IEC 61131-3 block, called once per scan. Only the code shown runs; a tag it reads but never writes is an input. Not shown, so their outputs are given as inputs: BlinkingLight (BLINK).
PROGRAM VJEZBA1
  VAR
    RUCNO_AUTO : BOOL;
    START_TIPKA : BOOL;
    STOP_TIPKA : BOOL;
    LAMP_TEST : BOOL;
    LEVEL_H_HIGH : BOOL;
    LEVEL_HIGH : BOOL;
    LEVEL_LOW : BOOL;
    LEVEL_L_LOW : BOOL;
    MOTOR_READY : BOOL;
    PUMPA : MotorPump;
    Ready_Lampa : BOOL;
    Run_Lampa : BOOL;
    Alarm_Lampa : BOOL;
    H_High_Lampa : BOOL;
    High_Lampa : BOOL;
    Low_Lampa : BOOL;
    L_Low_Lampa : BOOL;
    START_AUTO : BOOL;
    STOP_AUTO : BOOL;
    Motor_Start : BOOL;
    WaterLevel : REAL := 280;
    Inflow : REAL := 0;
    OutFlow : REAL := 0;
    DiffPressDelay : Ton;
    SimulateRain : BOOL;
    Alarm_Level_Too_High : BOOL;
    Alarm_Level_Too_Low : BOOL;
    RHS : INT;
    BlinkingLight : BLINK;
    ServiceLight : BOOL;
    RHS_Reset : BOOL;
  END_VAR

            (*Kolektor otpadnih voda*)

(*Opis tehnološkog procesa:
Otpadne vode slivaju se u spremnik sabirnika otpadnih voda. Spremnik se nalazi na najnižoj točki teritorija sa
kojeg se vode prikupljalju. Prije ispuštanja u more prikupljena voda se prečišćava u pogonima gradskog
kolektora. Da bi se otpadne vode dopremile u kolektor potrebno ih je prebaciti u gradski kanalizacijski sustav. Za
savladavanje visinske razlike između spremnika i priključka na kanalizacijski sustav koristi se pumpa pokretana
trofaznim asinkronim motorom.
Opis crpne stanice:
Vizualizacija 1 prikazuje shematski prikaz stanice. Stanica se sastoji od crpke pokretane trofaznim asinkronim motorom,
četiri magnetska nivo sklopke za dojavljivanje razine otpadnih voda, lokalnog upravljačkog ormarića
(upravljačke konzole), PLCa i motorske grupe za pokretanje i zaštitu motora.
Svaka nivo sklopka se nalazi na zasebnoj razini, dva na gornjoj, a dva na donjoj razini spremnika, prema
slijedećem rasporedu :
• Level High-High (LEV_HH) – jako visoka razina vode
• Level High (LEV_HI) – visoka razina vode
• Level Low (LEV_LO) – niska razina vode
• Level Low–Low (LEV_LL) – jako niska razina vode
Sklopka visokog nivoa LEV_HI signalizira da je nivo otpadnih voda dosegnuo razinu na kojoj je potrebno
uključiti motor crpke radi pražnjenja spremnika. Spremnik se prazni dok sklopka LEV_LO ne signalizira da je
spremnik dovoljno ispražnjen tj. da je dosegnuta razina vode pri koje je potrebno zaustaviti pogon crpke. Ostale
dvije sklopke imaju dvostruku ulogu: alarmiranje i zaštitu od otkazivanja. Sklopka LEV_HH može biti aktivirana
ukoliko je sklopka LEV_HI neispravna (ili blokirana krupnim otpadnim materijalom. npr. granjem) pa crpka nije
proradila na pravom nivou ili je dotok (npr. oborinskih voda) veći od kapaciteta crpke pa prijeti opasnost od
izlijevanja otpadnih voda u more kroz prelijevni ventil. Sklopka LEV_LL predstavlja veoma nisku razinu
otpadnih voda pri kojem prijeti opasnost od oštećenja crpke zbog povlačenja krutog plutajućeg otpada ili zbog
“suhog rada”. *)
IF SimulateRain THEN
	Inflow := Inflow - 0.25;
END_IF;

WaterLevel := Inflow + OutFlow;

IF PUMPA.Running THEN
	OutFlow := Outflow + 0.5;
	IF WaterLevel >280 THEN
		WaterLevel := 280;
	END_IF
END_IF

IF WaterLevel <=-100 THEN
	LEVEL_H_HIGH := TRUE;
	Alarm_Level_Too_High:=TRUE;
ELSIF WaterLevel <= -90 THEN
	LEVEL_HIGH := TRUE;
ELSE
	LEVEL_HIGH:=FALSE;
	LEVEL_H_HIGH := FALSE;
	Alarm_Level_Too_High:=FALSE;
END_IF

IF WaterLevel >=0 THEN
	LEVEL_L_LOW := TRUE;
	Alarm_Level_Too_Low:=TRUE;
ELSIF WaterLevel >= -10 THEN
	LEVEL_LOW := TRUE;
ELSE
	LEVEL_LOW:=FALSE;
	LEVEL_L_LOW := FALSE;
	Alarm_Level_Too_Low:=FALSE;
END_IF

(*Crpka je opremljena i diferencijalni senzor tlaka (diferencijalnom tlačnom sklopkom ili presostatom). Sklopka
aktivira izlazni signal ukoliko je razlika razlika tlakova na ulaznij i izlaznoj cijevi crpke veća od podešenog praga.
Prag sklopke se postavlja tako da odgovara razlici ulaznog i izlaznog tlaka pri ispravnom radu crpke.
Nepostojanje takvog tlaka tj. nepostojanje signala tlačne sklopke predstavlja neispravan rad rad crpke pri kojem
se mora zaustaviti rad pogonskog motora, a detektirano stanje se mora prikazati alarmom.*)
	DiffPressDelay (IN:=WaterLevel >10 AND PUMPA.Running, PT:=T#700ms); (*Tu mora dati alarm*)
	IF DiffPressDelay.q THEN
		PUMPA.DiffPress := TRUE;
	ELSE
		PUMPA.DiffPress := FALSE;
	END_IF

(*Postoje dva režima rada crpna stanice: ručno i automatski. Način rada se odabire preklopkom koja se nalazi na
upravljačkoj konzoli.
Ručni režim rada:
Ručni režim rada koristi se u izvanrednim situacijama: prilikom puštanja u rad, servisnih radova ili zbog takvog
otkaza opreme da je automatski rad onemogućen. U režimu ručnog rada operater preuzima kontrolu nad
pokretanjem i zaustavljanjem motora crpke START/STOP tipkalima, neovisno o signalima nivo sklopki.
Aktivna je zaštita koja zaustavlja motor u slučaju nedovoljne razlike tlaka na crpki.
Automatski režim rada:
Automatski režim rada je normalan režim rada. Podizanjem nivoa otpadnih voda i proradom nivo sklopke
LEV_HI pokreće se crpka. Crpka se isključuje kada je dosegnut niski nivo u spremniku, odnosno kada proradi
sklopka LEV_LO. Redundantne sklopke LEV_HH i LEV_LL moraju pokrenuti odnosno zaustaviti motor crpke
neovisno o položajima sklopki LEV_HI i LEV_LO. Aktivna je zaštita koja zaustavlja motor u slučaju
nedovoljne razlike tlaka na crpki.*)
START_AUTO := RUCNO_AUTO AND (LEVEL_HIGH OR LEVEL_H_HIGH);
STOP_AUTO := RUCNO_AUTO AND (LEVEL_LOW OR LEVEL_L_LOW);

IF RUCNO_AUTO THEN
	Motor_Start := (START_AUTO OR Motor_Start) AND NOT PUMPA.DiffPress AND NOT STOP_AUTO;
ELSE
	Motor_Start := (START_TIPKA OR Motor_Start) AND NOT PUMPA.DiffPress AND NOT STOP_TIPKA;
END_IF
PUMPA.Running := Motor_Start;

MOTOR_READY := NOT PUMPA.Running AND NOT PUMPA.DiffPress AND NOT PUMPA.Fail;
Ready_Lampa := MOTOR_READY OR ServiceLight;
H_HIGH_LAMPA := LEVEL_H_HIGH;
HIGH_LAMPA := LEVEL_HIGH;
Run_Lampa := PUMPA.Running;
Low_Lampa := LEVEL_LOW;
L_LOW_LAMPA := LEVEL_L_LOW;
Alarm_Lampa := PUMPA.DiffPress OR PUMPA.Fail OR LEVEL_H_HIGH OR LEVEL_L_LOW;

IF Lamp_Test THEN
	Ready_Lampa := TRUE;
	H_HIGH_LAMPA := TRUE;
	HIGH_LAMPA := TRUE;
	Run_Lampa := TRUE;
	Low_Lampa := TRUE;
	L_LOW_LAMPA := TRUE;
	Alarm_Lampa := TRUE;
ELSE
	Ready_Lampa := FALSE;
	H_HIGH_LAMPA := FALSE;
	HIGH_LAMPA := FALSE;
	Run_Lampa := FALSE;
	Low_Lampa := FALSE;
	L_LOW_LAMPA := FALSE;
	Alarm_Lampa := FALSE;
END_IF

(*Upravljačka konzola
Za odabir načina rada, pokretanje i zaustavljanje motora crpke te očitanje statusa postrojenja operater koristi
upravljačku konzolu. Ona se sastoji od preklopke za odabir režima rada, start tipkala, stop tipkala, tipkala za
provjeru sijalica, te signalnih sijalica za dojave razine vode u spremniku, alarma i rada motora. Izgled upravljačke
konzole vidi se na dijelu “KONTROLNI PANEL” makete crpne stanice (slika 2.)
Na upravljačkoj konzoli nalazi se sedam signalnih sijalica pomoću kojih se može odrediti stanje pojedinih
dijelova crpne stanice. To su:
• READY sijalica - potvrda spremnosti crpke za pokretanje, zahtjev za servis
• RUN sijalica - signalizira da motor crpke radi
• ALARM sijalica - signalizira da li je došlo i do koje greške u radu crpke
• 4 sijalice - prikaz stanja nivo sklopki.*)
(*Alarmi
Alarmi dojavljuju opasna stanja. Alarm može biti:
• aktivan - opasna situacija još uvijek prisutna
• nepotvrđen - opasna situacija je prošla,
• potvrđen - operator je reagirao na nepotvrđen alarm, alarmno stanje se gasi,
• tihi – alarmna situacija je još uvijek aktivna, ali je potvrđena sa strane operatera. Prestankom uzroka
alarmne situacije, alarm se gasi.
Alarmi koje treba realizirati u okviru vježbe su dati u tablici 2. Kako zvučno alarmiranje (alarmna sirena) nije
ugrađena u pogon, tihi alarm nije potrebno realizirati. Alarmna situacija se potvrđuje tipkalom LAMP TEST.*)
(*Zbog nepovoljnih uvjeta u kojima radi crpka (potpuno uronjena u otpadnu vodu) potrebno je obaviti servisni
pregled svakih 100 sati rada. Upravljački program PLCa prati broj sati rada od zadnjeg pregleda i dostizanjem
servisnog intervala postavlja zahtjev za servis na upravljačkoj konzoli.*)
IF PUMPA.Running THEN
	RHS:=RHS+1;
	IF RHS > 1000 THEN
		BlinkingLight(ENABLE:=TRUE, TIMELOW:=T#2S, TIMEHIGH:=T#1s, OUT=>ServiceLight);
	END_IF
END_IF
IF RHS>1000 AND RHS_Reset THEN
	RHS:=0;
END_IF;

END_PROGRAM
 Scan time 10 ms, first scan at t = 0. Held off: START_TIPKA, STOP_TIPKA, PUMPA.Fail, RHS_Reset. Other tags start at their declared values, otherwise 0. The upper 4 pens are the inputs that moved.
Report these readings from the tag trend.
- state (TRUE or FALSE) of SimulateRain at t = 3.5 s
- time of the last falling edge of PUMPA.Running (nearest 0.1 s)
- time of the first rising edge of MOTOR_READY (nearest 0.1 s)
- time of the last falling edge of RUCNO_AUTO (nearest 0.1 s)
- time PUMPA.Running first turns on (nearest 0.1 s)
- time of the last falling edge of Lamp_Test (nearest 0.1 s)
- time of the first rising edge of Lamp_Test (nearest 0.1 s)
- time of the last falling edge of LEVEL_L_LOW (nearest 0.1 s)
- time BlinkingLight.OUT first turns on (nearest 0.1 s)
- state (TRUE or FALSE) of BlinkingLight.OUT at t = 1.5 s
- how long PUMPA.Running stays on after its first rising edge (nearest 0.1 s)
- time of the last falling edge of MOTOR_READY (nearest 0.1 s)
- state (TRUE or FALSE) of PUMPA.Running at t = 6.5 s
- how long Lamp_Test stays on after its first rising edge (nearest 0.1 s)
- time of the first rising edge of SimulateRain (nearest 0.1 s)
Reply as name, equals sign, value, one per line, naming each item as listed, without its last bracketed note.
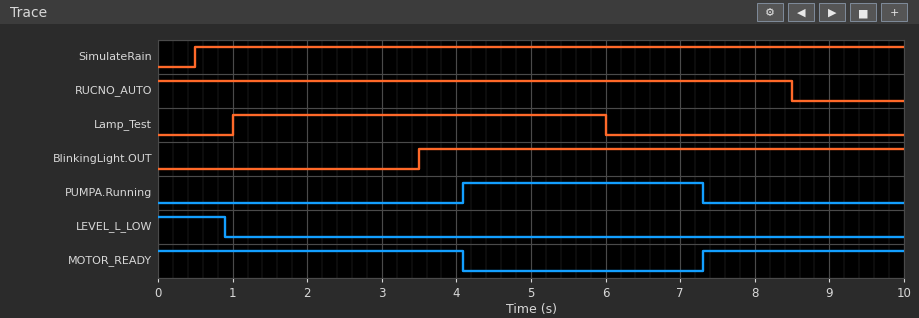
state (TRUE or FALSE) of SimulateRain at t = 3.5 s = TRUE
time of the last falling edge of PUMPA.Running = 7.3 s
time of the first rising edge of MOTOR_READY = 7.3 s
time of the last falling edge of RUCNO_AUTO = 8.5 s
time PUMPA.Running first turns on = 4.1 s
time of the last falling edge of Lamp_Test = 6.0 s
time of the first rising edge of Lamp_Test = 1.0 s
time of the last falling edge of LEVEL_L_LOW = 0.9 s
time BlinkingLight.OUT first turns on = 3.5 s
state (TRUE or FALSE) of BlinkingLight.OUT at t = 1.5 s = FALSE
how long PUMPA.Running stays on after its first rising edge = 3.2 s
time of the last falling edge of MOTOR_READY = 4.1 s
state (TRUE or FALSE) of PUMPA.Running at t = 6.5 s = TRUE
how long Lamp_Test stays on after its first rising edge = 5.0 s
time of the first rising edge of SimulateRain = 0.5 s
